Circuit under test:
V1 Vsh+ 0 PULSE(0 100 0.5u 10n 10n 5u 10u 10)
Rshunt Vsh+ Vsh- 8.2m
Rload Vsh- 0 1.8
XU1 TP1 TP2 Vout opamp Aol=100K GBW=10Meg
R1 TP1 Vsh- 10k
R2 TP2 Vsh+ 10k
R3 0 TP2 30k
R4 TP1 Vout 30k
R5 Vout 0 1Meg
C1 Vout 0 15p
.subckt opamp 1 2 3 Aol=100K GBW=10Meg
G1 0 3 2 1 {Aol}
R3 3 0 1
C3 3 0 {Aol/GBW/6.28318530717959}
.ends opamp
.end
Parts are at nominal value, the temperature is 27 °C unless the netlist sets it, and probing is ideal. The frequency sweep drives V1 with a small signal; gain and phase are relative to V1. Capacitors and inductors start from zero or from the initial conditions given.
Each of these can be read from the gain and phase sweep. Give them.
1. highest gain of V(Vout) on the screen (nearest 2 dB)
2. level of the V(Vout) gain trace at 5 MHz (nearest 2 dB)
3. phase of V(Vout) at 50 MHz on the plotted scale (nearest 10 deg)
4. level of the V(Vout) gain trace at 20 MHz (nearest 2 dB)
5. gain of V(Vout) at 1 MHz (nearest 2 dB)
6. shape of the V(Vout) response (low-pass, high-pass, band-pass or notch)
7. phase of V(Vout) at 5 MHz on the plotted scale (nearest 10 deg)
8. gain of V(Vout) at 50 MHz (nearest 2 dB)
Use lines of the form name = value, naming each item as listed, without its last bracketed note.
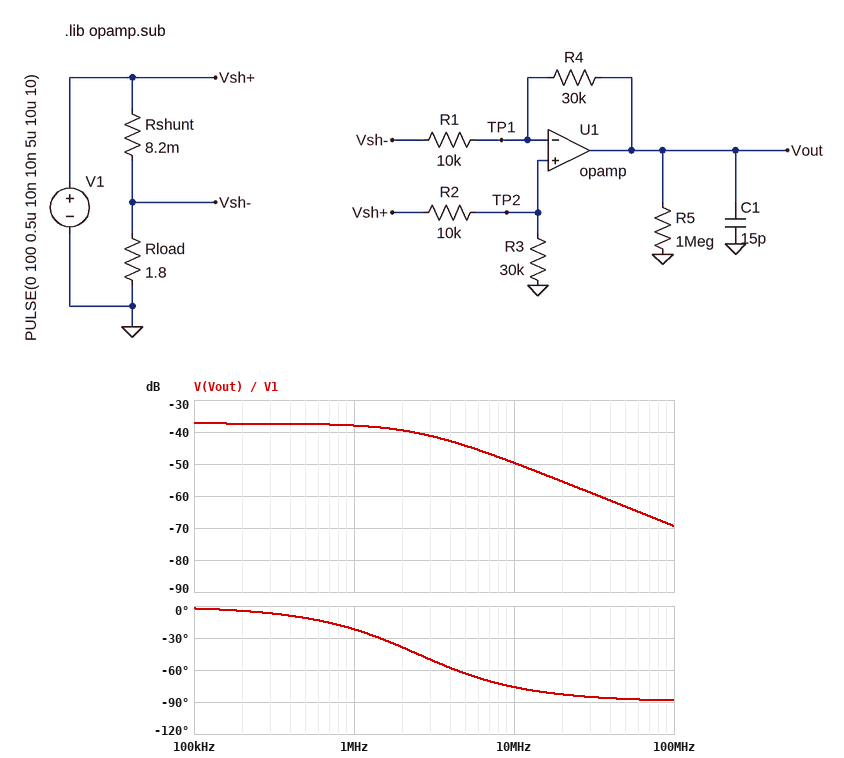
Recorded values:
highest gain of V(Vout) on the screen = -38 dB
level of the V(Vout) gain trace at 5 MHz = -44 dB
phase of V(Vout) at 50 MHz on the plotted scale = -90 deg
level of the V(Vout) gain trace at 20 MHz = -56 dB
gain of V(Vout) at 1 MHz = -38 dB
shape of the V(Vout) response = low-pass
phase of V(Vout) at 5 MHz on the plotted scale = -60 deg
gain of V(Vout) at 50 MHz = -64 dB
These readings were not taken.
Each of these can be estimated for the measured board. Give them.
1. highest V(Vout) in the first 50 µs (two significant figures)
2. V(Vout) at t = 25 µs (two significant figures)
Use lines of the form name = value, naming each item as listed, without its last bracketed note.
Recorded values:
highest V(Vout) in the first 50 µs = 1.4 V
V(Vout) at t = 25 µs = 1.4 V
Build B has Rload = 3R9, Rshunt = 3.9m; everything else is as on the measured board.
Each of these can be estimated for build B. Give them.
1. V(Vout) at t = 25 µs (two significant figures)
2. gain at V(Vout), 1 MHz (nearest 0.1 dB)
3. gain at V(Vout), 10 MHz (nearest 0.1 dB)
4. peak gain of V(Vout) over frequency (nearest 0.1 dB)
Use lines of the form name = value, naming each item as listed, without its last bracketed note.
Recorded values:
V(Vout) at t = 25 µs = 300 mV
gain at V(Vout), 1 MHz = -51.1 dB
gain at V(Vout), 10 MHz = -62.8 dB
peak gain of V(Vout) over frequency = -50.5 dB
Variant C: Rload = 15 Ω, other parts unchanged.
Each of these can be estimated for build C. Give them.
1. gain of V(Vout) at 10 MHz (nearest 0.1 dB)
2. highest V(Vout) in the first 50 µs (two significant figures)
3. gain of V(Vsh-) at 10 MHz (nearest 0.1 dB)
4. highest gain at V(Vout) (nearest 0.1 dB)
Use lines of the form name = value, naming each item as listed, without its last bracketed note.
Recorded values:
gain of V(Vout) at 10 MHz = -68.0 dB
highest V(Vout) in the first 50 µs = 160 mV
gain of V(Vsh-) at 10 MHz = 0 dB
highest gain at V(Vout) = -55.7 dB
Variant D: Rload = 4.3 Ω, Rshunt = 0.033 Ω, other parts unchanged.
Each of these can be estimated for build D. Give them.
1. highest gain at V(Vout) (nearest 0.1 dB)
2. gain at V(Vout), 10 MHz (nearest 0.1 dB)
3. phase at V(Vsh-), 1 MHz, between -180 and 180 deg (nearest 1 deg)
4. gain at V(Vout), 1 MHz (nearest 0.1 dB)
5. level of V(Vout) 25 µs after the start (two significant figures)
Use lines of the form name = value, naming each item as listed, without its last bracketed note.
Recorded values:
highest gain at V(Vout) = -32.8 dB
gain at V(Vout), 10 MHz = -45.1 dB
phase at V(Vsh-), 1 MHz, between -180 and 180 deg = 0 deg
gain at V(Vout), 1 MHz = -33.5 dB
level of V(Vout) 25 µs after the start = 2.3 V
